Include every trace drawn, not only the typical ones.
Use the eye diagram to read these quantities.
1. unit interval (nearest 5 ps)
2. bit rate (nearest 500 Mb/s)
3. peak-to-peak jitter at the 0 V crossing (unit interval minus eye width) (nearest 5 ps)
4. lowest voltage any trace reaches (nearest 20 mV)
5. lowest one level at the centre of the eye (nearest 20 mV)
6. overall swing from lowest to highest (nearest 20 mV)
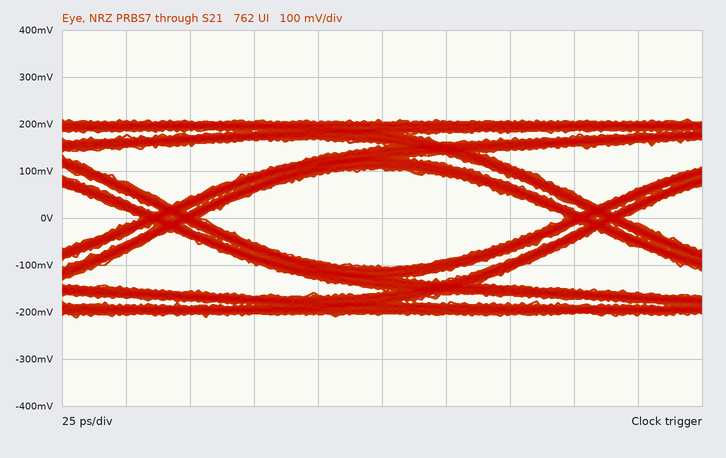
165 ps
6.0 Gb/s
25 ps
-220 mV
100 mV
420 mV
